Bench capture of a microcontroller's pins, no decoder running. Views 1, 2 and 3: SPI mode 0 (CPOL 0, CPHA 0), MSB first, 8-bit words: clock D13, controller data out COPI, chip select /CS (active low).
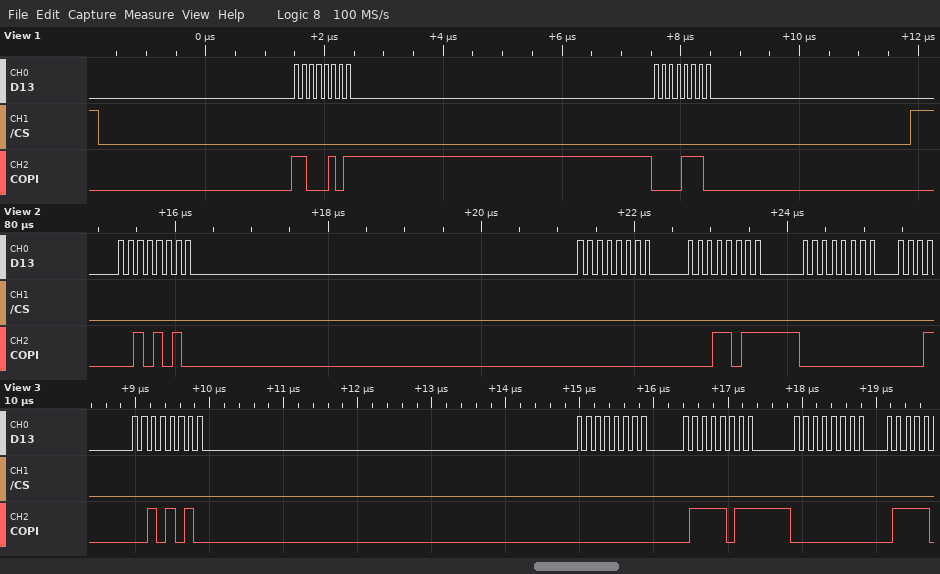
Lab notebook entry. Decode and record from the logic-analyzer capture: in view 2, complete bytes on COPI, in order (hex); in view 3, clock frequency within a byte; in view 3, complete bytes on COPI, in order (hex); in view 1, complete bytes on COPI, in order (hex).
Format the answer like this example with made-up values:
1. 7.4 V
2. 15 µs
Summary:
1. 0x2A 0x00 0x1B 0x00
2. 8 MHz
3. 2A 00 7B 00
4. C5 0E
